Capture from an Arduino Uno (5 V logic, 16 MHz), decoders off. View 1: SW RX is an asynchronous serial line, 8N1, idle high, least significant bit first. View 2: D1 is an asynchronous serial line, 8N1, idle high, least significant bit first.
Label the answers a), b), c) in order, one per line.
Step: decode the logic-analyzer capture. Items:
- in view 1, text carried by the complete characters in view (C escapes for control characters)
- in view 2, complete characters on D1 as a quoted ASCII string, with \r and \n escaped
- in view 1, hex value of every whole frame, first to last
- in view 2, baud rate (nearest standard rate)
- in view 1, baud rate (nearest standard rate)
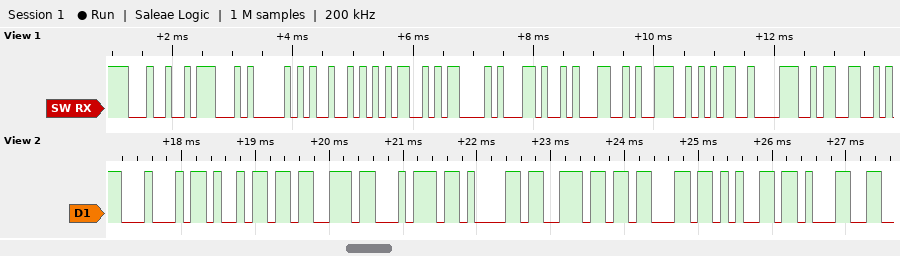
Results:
a) "$GPRMC,19583"
b) "Distance1"
c) 0x24 0x47 0x50 0x52 0x4D 0x43 0x2C 0x31 0x39 0x35 0x38 0x33
d) 9600 baud
e) 9600 baud
